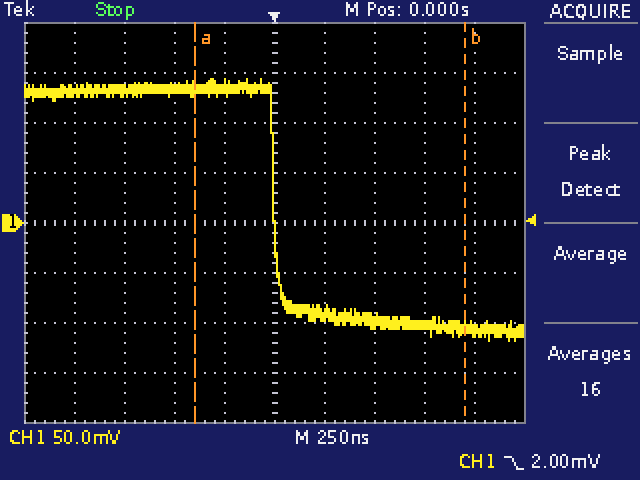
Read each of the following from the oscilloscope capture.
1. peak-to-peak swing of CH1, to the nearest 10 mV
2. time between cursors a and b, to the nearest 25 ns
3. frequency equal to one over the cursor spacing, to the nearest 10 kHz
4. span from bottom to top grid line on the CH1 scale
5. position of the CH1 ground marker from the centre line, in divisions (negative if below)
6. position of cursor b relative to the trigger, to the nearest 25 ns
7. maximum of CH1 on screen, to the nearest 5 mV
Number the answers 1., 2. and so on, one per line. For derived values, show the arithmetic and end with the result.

1. 260 mV
2. 1.350 µs
3. 1 / 1.350 µs ≈ 740 kHz
4. 400 mV
5. 0.0 div
6. +950 ns
7. 145 mV
